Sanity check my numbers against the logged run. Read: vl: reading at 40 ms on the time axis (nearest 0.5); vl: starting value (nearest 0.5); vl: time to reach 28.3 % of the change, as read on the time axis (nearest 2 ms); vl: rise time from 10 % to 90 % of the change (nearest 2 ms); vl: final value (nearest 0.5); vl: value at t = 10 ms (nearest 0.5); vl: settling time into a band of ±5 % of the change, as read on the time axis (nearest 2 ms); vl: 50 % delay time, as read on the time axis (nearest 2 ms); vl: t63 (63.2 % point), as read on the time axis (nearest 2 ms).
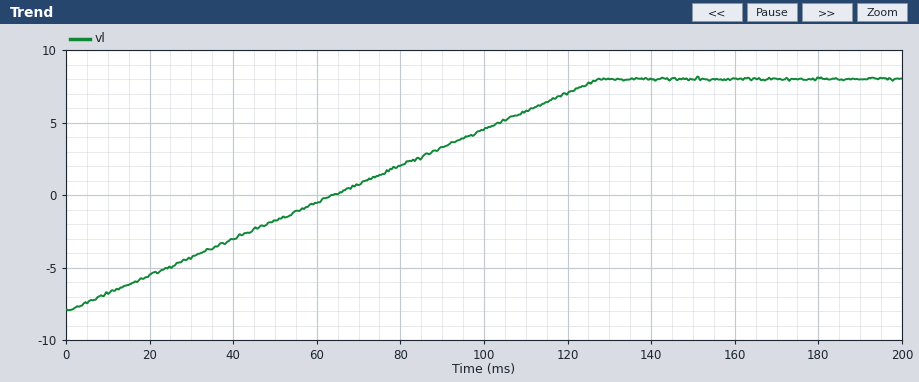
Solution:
-3.0
-8.0
36 ms
102 ms
8.0
-7.0
122 ms
64 ms
80 ms
